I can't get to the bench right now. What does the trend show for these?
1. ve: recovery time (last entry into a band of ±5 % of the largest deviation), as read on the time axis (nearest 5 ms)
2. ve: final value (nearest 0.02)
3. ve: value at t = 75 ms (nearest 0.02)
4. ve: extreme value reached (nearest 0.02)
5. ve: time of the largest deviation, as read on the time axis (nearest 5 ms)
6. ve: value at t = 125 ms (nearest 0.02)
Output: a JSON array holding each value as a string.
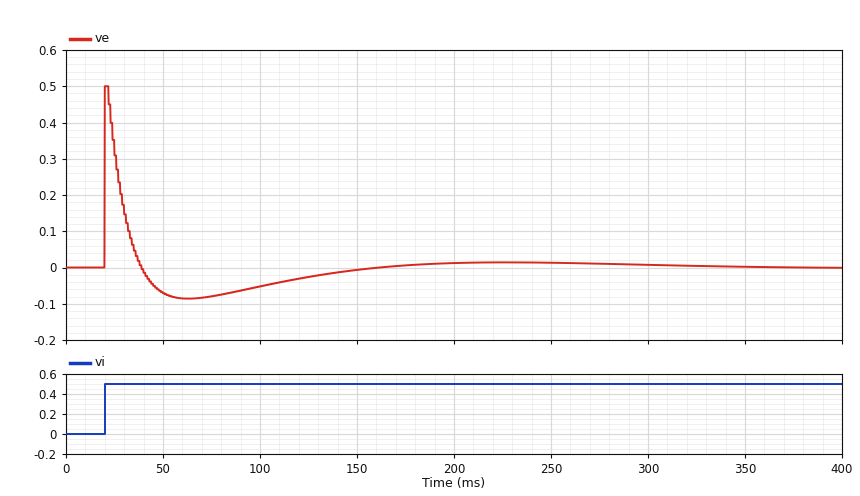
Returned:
["125 ms", "0.00", "-0.08", "0.50", "20 ms", "-0.02"]
